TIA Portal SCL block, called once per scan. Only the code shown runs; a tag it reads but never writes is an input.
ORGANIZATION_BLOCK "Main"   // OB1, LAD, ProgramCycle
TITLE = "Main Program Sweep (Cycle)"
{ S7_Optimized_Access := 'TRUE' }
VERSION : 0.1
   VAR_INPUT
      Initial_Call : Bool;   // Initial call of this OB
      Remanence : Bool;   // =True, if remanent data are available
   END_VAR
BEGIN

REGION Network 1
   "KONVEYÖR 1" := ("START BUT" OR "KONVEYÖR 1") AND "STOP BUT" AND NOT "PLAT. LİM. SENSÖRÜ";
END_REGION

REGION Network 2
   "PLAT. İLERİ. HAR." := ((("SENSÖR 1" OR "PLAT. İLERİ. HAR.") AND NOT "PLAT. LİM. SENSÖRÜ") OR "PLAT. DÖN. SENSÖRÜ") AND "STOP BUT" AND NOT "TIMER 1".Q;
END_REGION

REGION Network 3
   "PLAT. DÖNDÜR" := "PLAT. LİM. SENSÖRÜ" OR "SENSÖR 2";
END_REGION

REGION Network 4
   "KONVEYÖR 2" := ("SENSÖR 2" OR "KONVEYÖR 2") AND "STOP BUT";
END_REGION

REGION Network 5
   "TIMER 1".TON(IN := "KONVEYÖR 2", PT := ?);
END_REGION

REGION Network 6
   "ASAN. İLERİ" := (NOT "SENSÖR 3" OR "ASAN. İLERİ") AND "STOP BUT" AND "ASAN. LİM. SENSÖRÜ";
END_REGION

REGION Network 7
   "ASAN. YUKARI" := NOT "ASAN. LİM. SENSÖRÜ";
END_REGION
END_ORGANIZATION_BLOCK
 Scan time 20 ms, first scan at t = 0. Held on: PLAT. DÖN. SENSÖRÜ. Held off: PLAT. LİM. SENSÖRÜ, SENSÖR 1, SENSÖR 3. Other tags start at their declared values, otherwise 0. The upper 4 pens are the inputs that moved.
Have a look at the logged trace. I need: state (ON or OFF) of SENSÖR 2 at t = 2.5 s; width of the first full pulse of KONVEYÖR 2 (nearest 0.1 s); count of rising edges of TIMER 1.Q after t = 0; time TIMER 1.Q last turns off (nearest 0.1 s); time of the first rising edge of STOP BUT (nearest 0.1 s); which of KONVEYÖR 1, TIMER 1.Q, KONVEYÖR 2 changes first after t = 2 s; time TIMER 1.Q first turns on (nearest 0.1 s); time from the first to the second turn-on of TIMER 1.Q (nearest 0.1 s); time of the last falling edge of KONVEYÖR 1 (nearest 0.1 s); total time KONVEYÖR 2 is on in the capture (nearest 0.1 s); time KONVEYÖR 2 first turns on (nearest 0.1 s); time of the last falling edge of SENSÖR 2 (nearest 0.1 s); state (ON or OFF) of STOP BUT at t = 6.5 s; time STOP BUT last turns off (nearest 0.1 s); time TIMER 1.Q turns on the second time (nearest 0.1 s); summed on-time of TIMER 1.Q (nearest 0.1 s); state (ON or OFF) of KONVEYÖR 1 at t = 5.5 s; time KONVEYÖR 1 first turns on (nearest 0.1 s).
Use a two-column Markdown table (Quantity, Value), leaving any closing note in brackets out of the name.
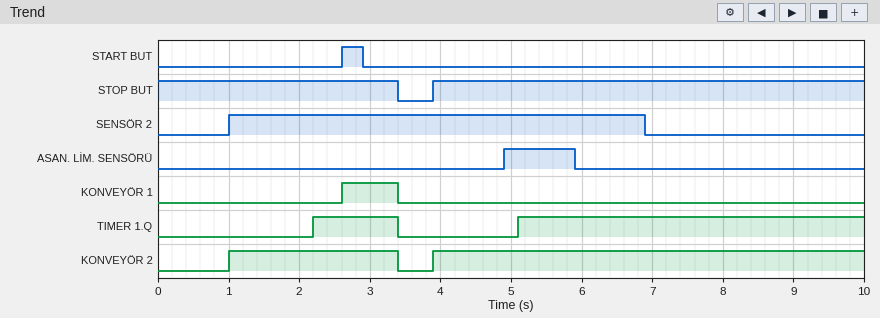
| Quantity | Value |
|---|---|
| state (ON or OFF) of SENSÖR 2 at t = 2.5 s | ON |
| width of the first full pulse of KONVEYÖR 2 | 2.4 s |
| count of rising edges of TIMER 1.Q after t = 0 | 2 |
| time TIMER 1.Q last turns off | 3.4 s |
| time of the first rising edge of STOP BUT | 3.9 s |
| which of KONVEYÖR 1, TIMER 1.Q, KONVEYÖR 2 changes first after t = 2 s | TIMER 1.Q |
| time TIMER 1.Q first turns on | 2.2 s |
| time from the first to the second turn-on of TIMER 1.Q | 2.9 s |
| time of the last falling edge of KONVEYÖR 1 | 3.4 s |
| total time KONVEYÖR 2 is on in the capture | 8.5 s |
| time KONVEYÖR 2 first turns on | 1.0 s |
| time of the last falling edge of SENSÖR 2 | 6.9 s |
| state (ON or OFF) of STOP BUT at t = 6.5 s | ON |
| time STOP BUT last turns off | 3.4 s |
| time TIMER 1.Q turns on the second time | 5.1 s |
| summed on-time of TIMER 1.Q | 6.1 s |
| state (ON or OFF) of KONVEYÖR 1 at t = 5.5 s | OFF |
| time KONVEYÖR 1 first turns on | 2.6 s |
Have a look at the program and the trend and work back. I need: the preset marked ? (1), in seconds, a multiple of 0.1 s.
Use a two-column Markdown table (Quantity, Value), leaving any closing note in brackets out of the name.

| Quantity | Value |
|---|---|
| the preset marked ? (1), in seconds, a multiple of 0.1 s | 1.2 s |
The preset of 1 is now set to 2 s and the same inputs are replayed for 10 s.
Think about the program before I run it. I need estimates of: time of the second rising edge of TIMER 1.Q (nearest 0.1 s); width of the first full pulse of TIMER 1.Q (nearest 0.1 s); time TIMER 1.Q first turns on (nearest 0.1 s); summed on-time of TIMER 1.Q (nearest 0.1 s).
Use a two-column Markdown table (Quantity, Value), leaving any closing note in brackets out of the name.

| Quantity | Value |
|---|---|
| time of the second rising edge of TIMER 1.Q | 5.9 s |
| width of the first full pulse of TIMER 1.Q | 0.4 s |
| time TIMER 1.Q first turns on | 3.0 s |
| summed on-time of TIMER 1.Q | 4.5 s |
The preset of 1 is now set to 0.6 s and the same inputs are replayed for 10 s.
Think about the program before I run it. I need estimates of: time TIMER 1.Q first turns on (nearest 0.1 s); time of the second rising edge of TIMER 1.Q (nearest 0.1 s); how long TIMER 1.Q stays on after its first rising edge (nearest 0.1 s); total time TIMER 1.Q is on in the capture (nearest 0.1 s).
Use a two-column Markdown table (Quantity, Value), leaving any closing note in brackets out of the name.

| Quantity | Value |
|---|---|
| time TIMER 1.Q first turns on | 1.6 s |
| time of the second rising edge of TIMER 1.Q | 4.5 s |
| how long TIMER 1.Q stays on after its first rising edge | 1.8 s |
| total time TIMER 1.Q is on in the capture | 7.3 s |
